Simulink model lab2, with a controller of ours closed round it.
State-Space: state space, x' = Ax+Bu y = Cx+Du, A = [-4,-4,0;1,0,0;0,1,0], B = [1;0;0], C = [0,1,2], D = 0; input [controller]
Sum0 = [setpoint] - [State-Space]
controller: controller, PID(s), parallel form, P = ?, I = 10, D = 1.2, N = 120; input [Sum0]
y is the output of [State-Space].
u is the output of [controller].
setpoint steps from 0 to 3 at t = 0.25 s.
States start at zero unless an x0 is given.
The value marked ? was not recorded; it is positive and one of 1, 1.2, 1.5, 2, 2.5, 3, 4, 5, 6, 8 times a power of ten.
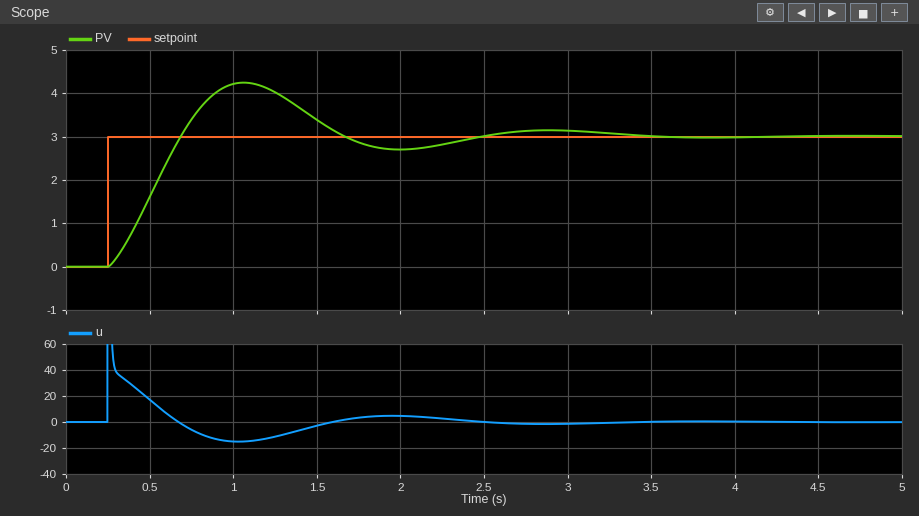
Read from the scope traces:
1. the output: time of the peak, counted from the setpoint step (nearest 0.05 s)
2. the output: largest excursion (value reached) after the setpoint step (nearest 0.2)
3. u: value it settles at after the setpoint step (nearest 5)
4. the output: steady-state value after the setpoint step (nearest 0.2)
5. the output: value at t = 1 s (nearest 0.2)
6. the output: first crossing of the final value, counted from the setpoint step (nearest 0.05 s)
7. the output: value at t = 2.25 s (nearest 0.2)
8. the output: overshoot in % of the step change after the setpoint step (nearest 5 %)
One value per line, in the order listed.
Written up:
0.80 s
4.2
0
3.0
4.2
0.45 s
2.8
40 %
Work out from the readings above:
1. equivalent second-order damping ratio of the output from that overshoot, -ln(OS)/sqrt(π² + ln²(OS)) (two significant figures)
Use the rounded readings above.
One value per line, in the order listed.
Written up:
0.28
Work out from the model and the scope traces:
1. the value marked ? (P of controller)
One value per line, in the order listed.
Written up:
15
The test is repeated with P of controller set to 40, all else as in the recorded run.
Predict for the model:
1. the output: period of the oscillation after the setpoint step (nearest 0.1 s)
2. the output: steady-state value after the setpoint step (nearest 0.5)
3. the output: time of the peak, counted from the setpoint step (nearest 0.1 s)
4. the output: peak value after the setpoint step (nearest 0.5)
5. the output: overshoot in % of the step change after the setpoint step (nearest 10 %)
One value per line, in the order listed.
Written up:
1.0 s
3.0
0.5 s
4.5
50 %
